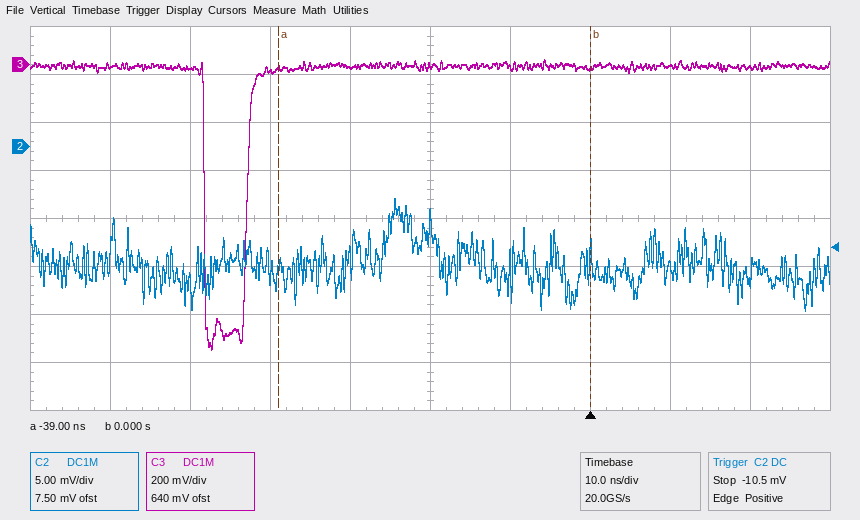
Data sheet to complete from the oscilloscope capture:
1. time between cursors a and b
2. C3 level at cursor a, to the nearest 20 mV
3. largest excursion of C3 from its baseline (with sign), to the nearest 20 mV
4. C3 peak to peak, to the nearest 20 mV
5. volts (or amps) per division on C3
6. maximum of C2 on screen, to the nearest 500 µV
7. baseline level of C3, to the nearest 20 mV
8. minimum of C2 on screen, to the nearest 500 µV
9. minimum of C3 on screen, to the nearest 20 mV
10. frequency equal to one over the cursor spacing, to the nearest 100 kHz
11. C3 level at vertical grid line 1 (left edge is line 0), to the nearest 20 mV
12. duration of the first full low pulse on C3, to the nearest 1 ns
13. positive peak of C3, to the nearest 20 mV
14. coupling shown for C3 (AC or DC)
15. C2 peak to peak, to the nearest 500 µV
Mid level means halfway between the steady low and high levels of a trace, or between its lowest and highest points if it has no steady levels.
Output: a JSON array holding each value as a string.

["39 ns", "-20 mV", "-1.18 V", "1.20 V", "200 mV", "-5.5 mV", "0 mV", "-17.0 mV", "-1.18 V", "25.6 MHz", "0 mV", "5 ns", "20 mV", "DC", "11.5 mV"]
